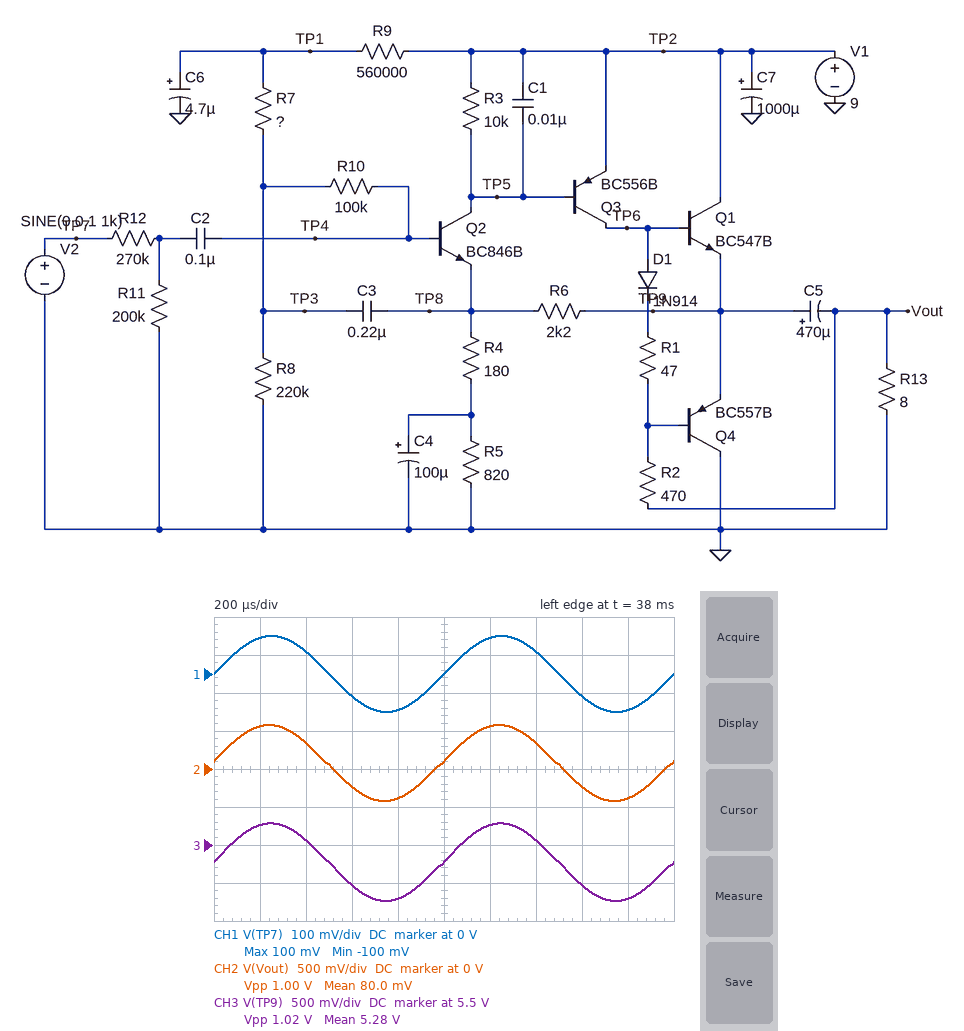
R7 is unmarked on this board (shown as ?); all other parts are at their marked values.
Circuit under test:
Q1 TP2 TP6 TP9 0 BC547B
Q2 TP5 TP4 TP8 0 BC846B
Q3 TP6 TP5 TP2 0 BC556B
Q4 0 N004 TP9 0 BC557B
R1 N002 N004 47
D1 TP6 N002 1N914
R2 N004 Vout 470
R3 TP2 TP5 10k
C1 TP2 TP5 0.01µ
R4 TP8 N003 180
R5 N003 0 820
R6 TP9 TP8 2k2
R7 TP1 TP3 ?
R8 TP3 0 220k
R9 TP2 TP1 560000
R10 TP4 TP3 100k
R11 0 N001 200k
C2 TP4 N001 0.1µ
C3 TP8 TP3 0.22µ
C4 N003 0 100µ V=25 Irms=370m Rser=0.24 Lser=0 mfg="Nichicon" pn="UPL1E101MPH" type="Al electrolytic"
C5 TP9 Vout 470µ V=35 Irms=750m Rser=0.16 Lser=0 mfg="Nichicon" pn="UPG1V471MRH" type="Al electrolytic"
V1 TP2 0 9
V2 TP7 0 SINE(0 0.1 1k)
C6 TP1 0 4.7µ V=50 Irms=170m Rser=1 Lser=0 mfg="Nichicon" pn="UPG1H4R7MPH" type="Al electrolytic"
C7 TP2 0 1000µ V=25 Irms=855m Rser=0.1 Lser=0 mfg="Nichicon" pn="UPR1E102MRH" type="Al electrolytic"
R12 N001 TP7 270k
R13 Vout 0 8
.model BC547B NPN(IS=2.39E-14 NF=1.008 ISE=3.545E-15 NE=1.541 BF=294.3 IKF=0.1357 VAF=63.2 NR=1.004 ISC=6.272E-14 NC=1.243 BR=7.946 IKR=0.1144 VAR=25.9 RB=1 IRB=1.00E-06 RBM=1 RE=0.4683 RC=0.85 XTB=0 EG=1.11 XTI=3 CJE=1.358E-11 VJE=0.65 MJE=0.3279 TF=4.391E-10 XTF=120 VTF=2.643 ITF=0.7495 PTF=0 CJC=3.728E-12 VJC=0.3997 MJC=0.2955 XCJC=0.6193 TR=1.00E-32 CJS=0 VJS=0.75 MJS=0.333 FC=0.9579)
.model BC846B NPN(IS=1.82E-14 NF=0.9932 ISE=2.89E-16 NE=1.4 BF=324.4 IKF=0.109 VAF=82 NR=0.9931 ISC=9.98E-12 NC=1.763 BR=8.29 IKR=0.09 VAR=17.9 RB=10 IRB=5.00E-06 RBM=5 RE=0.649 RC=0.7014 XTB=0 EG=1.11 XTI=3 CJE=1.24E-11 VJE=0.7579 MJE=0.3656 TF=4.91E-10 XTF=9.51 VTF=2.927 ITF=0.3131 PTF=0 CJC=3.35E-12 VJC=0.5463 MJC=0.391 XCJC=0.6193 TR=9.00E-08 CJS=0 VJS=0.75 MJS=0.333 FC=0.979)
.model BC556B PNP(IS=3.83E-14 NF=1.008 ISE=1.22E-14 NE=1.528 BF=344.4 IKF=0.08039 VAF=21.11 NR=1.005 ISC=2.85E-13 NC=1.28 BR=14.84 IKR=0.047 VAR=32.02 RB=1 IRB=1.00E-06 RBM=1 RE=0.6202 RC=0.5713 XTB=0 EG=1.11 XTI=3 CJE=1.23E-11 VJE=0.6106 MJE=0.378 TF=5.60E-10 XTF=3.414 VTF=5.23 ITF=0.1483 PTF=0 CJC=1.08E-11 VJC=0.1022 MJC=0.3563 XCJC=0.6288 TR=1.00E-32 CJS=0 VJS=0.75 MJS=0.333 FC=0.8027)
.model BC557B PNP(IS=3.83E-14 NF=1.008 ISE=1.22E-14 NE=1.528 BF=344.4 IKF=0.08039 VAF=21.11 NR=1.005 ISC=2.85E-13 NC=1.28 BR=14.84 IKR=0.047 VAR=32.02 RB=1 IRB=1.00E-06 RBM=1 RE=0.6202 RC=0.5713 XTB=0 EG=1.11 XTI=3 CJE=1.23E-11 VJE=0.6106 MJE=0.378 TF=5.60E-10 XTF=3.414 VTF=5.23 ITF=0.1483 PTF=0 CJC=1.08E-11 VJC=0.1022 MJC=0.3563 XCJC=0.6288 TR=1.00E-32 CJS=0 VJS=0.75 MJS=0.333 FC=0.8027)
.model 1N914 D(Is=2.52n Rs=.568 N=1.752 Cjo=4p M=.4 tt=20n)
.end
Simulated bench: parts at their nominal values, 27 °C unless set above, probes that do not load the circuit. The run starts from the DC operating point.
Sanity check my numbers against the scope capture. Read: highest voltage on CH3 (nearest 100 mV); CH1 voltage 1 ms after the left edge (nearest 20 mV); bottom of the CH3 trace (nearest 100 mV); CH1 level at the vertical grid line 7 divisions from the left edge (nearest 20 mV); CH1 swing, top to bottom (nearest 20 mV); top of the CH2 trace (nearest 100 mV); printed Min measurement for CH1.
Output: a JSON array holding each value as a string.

["5.8 V", "0 V", "4.8 V", "60 mV", "200 mV", "600 mV", "-100 mV"]
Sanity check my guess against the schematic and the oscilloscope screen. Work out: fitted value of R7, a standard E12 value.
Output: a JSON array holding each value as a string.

["56 kΩ"]
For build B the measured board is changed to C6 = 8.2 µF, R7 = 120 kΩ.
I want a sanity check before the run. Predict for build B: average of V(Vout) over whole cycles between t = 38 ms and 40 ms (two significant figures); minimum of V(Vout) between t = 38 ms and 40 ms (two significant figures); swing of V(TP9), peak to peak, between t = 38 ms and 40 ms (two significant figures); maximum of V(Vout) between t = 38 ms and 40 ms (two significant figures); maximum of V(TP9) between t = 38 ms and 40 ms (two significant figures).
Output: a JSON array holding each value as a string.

["70 mV", "-430 mV", "1.0 V", "570 mV", "5.3 V"]
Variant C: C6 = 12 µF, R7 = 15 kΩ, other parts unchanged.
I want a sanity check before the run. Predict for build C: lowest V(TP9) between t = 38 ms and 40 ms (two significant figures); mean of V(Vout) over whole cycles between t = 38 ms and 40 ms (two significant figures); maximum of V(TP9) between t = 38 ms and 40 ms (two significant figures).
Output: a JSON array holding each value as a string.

["5.1 V", "85 mV", "6.2 V"]
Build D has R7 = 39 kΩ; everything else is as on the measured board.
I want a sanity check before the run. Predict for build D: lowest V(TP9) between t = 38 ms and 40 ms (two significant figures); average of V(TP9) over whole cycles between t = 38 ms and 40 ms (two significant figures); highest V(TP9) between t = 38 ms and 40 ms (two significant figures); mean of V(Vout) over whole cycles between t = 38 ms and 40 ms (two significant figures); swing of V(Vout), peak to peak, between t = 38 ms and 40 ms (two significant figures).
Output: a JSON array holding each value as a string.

["4.9 V", "5.4 V", "5.9 V", "81 mV", "1.0 V"]
